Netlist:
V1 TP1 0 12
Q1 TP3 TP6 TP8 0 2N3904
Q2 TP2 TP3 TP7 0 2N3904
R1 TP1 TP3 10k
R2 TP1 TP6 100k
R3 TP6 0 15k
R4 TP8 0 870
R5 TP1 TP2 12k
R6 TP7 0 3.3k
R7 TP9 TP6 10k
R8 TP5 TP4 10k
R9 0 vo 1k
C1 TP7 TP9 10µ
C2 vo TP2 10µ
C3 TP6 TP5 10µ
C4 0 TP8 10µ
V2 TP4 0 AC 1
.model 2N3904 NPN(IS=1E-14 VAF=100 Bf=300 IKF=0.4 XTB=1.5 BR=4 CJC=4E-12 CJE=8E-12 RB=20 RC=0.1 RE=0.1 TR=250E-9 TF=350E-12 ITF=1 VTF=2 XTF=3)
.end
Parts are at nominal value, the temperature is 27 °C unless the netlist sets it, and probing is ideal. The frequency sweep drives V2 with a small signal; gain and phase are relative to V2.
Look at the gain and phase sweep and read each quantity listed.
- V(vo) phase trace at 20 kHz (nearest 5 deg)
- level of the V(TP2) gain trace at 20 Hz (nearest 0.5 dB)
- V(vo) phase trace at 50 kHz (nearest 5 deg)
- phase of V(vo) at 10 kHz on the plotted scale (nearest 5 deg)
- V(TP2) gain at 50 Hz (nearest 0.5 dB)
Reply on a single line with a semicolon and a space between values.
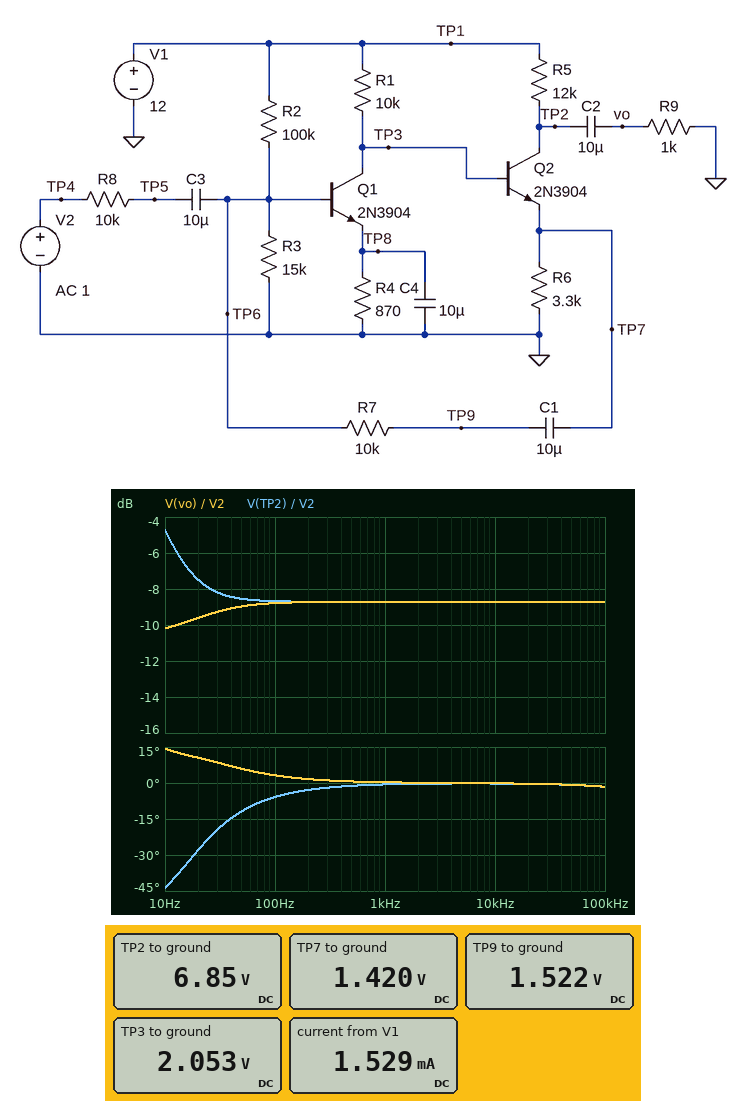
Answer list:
0 deg; -7.5 dB; 0 deg; 0 deg; -8.5 dB
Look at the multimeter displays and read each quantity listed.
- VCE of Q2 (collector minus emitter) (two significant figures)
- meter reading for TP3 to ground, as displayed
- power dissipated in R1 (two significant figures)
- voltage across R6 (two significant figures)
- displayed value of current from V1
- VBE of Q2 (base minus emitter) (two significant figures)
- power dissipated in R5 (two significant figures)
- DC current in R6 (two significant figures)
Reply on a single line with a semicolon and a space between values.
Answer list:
5.4 V; 2.053 V; 9.9 mW; 1.4 V; 1.529 mA; 630 mV; 2.2 mW; 430 µA
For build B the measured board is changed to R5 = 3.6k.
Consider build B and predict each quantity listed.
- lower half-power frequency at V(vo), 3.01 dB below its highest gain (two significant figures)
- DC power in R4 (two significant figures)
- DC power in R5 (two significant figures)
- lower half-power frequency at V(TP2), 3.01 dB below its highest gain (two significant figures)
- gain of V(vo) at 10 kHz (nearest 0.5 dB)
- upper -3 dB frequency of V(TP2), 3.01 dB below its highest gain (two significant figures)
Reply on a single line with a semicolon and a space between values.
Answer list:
5.8 Hz; 860 µW; 660 µW; 110 mHz; -10.0 dB; 5.4 Hz
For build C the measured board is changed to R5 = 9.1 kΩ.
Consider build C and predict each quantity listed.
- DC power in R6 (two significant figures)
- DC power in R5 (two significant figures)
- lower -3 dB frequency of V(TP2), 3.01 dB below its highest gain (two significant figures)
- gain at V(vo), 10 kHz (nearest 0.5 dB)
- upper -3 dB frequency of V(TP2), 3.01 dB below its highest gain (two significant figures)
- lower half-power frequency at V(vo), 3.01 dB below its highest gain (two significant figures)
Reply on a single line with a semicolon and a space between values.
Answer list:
610 µW; 1.7 mW; 90 mHz; -9.0 dB; 2.5 Hz; 3.2 Hz
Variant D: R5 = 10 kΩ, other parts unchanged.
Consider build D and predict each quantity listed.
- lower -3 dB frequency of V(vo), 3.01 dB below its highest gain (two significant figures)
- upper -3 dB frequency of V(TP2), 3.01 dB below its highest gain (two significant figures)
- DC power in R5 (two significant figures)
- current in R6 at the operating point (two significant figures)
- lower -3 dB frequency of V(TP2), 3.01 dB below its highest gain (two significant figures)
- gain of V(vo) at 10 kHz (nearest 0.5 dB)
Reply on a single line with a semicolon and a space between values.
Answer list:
3.0 Hz; 2.3 Hz; 1.8 mW; 430 µA; 89 mHz; -9.0 dB
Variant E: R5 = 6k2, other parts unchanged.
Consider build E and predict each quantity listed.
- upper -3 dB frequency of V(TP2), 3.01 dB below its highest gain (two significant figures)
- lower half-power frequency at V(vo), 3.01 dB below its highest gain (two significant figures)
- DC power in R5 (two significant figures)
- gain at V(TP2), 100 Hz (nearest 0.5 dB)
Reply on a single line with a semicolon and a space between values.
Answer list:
3.5 Hz; 4.1 Hz; 1.1 mW; -9.5 dB
